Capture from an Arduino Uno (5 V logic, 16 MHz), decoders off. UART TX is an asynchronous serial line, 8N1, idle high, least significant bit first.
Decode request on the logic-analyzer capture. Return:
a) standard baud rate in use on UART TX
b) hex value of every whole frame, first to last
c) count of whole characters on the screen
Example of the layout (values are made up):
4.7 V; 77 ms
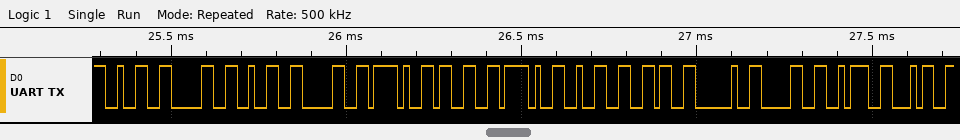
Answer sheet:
57600 baud; 0x32 0x30 0x32 0x30 0x2F 0x33 0x2F 0x32 0x36 0x20 0x30 0x3A 0x34; 13
